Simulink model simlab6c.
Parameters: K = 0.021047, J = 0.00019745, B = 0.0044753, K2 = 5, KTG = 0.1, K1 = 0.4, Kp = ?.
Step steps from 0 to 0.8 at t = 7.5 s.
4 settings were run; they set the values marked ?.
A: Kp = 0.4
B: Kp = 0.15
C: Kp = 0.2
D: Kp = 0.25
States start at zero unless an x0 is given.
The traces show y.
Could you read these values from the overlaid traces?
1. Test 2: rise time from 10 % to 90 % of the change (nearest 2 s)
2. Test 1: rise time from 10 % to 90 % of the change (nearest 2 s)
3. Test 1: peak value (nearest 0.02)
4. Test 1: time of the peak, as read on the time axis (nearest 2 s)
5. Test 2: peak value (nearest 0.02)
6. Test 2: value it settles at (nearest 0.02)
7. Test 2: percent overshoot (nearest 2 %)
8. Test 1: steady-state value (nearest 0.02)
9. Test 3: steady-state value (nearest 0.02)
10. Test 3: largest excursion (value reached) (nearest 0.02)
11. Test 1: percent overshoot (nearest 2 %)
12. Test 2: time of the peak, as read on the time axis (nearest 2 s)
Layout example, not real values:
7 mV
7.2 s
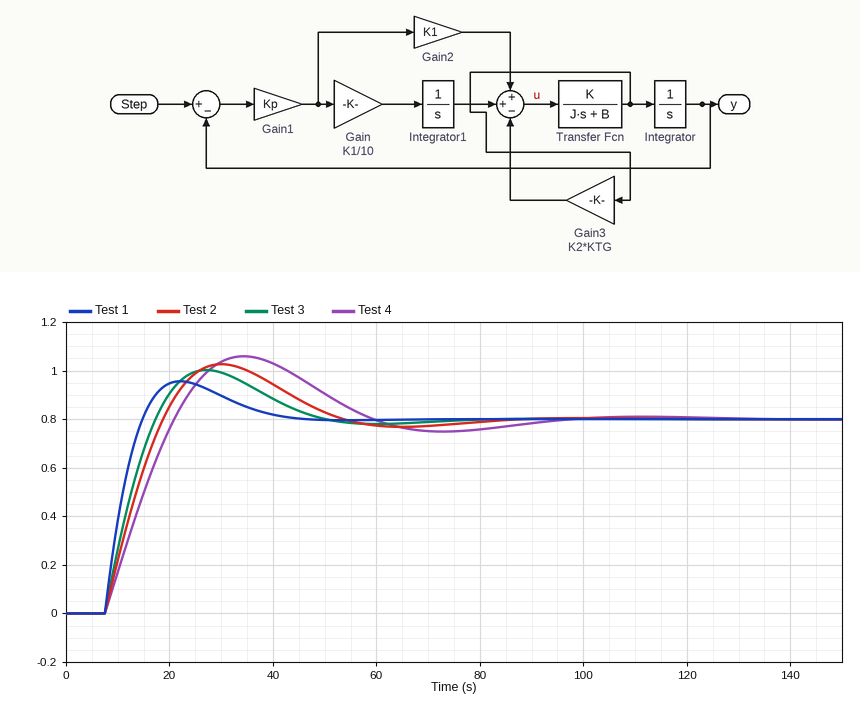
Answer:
8 s
6 s
0.96
22 s
1.02
0.80
28 %
0.80
0.80
1.00
20 %
30 s
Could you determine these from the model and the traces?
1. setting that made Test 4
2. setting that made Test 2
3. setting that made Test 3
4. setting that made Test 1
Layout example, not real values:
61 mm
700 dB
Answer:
B
C
D
A
